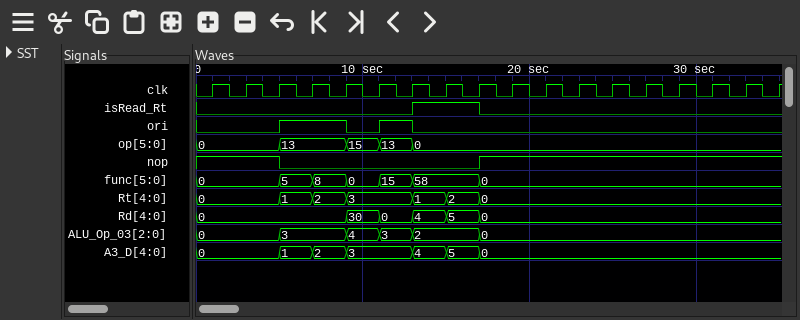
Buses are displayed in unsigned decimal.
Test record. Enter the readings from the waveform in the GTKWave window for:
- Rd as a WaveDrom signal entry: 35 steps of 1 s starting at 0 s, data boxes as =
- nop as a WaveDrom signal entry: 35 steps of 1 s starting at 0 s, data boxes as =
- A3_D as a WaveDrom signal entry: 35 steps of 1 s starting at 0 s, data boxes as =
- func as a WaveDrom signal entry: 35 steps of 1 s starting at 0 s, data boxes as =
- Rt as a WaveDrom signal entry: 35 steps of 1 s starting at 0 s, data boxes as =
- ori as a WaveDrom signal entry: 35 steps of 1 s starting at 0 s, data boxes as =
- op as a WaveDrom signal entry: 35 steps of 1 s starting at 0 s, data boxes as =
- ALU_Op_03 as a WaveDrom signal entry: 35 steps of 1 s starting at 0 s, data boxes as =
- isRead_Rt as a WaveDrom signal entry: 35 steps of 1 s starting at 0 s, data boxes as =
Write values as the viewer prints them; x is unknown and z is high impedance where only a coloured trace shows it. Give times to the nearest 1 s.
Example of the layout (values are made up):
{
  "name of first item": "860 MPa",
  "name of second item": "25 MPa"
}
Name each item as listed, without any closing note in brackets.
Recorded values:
{
  "Rd as a WaveDrom signal entry: 35 steps of 1 s starting at 0 s, data boxes as =": "{name: 'Rd', wave: '=........=.=.=.=.=.................', data: '0 30 0 4 5 0'}",
  "nop as a WaveDrom signal entry: 35 steps of 1 s starting at 0 s, data boxes as =": "{name: 'nop', wave: '1....0...........1.................'}",
  "A3_D as a WaveDrom signal entry: 35 steps of 1 s starting at 0 s, data boxes as =": "{name: 'A3_D', wave: '=....=.=.=...=.=.=.................', data: '0 1 2 3 4 5 0'}",
  "func as a WaveDrom signal entry: 35 steps of 1 s starting at 0 s, data boxes as =": "{name: 'func', wave: '=....=.=.=.=.=...=.................', data: '0 5 8 0 15 58 0'}",
  "Rt as a WaveDrom signal entry: 35 steps of 1 s starting at 0 s, data boxes as =": "{name: 'Rt', wave: '=....=.=.=...=.=.=.................', data: '0 1 2 3 1 2 0'}",
  "ori as a WaveDrom signal entry: 35 steps of 1 s starting at 0 s, data boxes as =": "{name: 'ori', wave: '0....1...0.1.0.....................'}",
  "op as a WaveDrom signal entry: 35 steps of 1 s starting at 0 s, data boxes as =": "{name: 'op', wave: '=....=...=.=.=.....................', data: '0 13 15 13 0'}",
  "ALU_Op_03 as a WaveDrom signal entry: 35 steps of 1 s starting at 0 s, data boxes as =": "{name: 'ALU_Op_03', wave: '=....=...=.=.=...=.................', data: '0 3 4 3 2 0'}",
  "isRead_Rt as a WaveDrom signal entry: 35 steps of 1 s starting at 0 s, data boxes as =": "{name: 'isRead_Rt', wave: '0............1...0.................'}"
}
